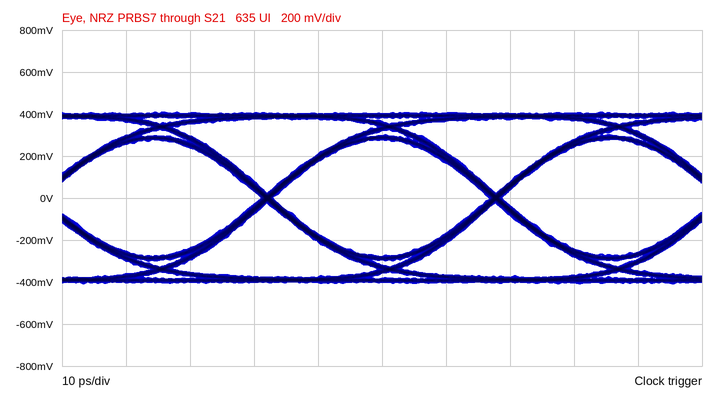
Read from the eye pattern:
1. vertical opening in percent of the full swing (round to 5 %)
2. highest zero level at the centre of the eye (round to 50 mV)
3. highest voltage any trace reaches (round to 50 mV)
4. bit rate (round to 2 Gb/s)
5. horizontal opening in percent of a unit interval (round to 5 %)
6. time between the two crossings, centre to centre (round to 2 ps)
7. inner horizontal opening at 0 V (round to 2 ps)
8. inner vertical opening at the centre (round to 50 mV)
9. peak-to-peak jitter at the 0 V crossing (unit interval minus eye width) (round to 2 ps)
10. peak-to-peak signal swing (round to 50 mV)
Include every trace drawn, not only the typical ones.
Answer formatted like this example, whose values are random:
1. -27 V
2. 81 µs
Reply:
1. 70 %
2. -300 mV
3. 400 mV
4. 28 Gb/s
5. 95 %
6. 36 ps
7. 34 ps
8. 550 mV
9. 2 ps
10. 800 mV
